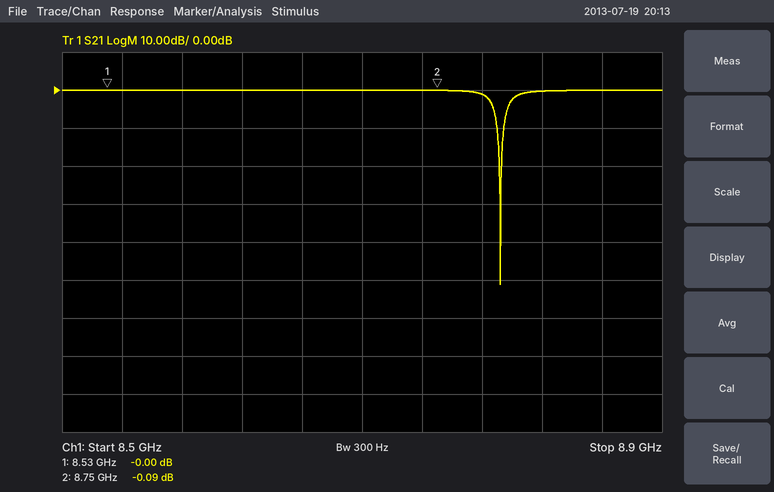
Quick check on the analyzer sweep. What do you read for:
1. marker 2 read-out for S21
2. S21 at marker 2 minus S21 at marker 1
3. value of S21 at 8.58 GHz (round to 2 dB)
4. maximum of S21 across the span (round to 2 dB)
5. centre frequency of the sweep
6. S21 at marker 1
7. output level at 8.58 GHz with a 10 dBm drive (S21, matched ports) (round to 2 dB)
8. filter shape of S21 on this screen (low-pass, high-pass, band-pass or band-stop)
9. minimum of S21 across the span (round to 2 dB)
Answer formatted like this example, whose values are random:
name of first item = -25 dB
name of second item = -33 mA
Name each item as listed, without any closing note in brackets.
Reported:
marker 2 read-out for S21 = -0.09 dB
S21 at marker 2 minus S21 at marker 1 = -0.09 dB
value of S21 at 8.58 GHz = 0 dB
maximum of S21 across the span = 0 dB
centre frequency of the sweep = 8.7 GHz
S21 at marker 1 = -0.00 dB
output level at 8.58 GHz with a 10 dBm drive (S21, matched ports) = 10 dBm
filter shape of S21 on this screen = band-stop
minimum of S21 across the span = -52 dB
